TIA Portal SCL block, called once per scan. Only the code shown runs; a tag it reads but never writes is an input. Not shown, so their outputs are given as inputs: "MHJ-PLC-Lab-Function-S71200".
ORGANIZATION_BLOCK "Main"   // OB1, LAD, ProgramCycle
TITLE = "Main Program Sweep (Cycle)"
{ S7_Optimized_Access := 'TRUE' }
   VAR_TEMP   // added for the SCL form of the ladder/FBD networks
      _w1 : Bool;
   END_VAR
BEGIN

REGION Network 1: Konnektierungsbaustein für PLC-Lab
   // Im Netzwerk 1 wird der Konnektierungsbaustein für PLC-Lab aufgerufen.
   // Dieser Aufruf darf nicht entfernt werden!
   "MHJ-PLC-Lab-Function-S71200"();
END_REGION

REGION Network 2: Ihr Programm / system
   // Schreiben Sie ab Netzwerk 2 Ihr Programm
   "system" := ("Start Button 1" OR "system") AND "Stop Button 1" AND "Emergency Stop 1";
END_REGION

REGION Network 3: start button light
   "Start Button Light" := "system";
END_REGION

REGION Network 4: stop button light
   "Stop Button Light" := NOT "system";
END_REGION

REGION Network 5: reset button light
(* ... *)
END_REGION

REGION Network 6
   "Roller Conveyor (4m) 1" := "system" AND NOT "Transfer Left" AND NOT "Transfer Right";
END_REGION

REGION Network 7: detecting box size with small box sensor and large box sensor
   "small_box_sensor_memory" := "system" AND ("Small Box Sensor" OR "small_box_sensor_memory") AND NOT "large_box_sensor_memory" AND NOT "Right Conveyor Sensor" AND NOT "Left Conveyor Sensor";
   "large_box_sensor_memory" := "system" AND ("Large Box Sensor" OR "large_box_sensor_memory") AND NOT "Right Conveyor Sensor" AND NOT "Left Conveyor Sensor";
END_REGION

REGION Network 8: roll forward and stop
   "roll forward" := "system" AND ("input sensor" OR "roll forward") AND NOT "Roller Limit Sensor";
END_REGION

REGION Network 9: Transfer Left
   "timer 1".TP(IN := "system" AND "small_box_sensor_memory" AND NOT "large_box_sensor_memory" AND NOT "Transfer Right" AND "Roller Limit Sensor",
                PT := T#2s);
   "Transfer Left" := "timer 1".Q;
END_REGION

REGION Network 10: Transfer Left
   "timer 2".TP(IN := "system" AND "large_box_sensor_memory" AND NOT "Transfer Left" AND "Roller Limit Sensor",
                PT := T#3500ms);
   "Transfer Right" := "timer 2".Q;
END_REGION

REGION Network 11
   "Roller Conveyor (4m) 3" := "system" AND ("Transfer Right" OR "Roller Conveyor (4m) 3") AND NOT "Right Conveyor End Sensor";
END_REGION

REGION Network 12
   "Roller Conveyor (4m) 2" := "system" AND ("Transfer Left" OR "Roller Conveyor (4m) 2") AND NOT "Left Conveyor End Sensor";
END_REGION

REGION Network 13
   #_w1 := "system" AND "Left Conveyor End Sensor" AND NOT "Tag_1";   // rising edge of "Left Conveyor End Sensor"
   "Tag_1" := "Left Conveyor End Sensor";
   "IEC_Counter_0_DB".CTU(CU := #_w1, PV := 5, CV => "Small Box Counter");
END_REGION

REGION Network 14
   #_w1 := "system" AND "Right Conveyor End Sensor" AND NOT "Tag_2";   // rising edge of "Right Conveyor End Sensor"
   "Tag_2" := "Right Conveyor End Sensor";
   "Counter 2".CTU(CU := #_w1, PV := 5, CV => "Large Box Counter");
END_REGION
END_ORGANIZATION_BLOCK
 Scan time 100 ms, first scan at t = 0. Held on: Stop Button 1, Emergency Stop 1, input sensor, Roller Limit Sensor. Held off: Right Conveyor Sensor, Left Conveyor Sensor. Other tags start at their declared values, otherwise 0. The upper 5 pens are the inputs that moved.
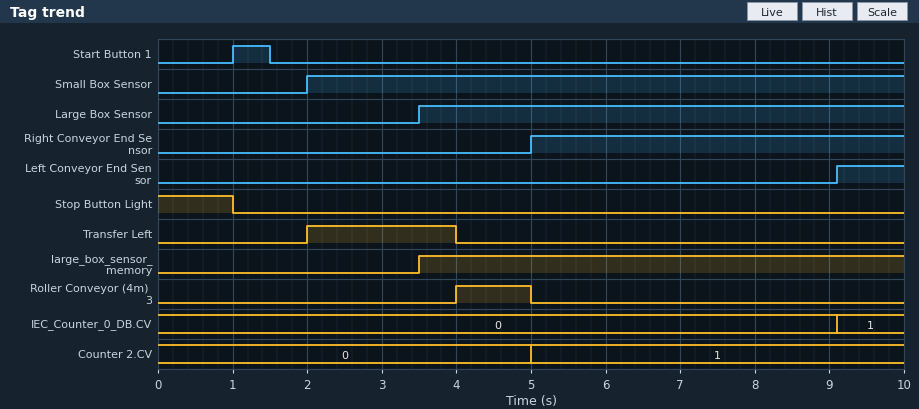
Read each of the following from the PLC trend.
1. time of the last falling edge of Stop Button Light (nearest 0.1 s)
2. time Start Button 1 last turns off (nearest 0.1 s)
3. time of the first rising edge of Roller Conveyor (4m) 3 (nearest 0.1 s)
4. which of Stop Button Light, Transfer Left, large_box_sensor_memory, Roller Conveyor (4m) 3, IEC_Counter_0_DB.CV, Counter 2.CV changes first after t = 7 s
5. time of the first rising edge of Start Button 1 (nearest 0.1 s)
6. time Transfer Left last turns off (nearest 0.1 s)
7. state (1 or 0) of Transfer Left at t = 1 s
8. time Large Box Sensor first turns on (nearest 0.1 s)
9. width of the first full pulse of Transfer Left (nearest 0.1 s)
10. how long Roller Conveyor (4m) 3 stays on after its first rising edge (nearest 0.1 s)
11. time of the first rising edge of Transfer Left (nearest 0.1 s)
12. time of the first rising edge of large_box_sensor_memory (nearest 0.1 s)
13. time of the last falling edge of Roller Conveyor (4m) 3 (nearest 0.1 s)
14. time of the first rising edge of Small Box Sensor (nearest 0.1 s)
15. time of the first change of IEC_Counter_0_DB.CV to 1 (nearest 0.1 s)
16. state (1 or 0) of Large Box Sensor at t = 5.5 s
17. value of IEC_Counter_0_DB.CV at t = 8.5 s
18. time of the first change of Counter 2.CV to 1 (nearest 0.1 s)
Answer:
1.0 s
1.5 s
4.0 s
IEC_Counter_0_DB.CV
1.0 s
4.0 s
0
3.5 s
2.0 s
1.0 s
2.0 s
3.5 s
5.0 s
2.0 s
9.1 s
1
0
5.0 s
